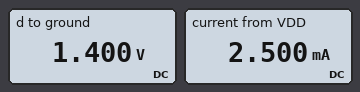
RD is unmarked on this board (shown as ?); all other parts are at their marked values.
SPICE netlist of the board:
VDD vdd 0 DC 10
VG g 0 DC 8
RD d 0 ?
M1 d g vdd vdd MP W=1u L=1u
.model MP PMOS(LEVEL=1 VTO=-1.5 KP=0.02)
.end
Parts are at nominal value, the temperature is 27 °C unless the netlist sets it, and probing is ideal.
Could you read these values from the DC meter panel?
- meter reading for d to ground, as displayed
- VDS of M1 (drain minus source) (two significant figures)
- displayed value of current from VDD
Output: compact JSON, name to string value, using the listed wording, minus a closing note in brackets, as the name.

{"meter reading for d to ground, as displayed": "1.400 V", "VDS of M1 (drain minus source)": "-8.6 V", "displayed value of current from VDD": "2.500 mA"}
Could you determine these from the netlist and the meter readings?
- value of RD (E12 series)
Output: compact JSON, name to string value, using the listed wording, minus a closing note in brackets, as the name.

{"value of RD": "560 Ω"}
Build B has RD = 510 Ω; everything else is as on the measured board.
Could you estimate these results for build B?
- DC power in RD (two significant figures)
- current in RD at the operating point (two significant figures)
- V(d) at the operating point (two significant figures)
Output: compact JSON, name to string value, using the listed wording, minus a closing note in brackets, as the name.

{"DC power in RD": "3.2 mW", "current in RD at the operating point": "2.5 mA", "V(d) at the operating point": "1.3 V"}
